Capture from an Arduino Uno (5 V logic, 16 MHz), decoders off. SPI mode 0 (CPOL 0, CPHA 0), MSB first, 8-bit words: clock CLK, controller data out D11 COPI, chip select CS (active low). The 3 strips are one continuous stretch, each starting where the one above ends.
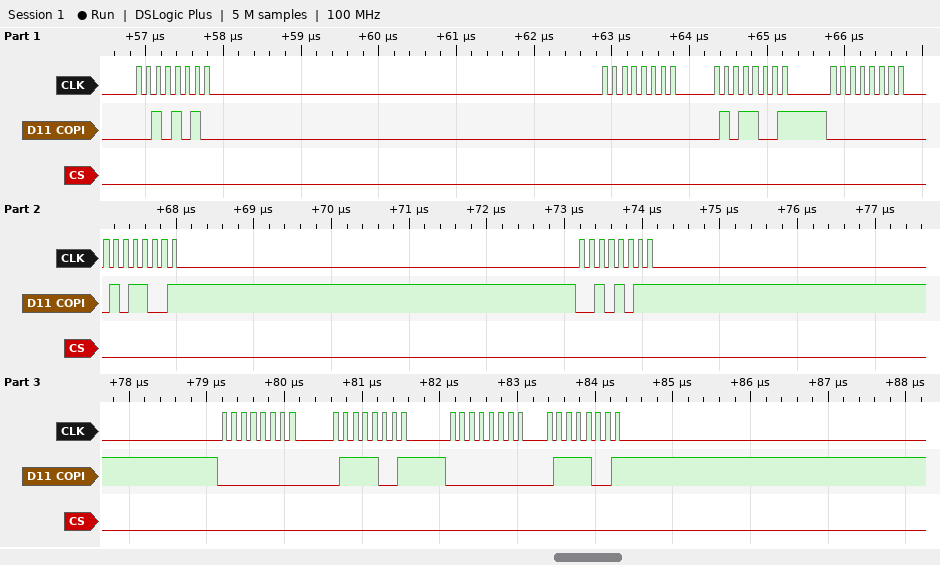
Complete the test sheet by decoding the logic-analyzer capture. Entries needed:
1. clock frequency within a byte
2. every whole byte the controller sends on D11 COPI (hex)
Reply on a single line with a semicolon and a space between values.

8 MHz; 2A 00 59 00 59 2B 00 79 00 79
